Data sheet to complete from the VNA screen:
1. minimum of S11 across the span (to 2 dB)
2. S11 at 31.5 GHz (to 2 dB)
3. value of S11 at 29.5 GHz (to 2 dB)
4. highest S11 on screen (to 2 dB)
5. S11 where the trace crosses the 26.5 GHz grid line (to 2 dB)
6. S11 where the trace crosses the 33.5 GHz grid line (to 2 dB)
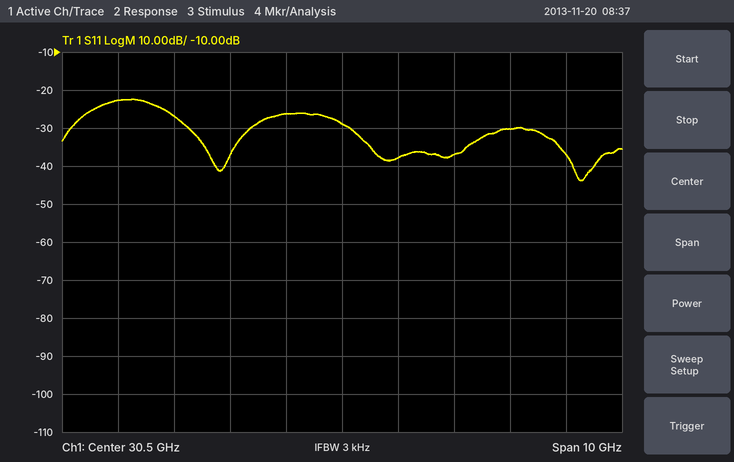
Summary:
-44 dB
-38 dB
-26 dB
-22 dB
-22 dB
-30 dB
